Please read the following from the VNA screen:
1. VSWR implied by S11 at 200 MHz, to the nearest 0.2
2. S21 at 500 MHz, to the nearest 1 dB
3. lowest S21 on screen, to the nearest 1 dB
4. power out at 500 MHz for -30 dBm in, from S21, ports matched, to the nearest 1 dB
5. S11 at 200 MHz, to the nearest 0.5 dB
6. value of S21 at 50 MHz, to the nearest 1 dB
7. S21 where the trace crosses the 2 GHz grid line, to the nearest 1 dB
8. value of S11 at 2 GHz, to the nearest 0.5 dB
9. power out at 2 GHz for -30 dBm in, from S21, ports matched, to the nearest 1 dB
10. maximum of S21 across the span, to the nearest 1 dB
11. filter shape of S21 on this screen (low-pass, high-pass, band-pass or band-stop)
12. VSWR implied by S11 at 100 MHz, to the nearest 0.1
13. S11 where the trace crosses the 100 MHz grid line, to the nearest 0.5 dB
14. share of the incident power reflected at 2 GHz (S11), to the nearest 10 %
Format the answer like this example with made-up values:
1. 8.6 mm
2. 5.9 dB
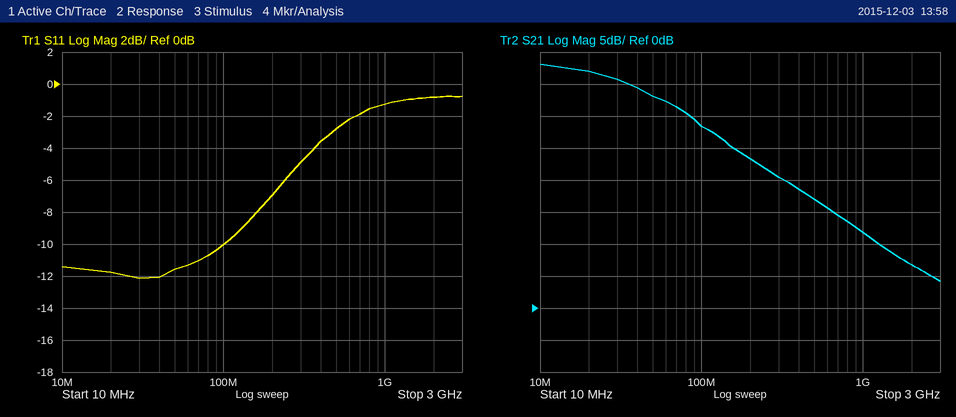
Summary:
1. 2.6
2. 17 dB
3. 4 dB
4. -13 dBm
5. -7.0 dB
6. 33 dB
7. 7 dB
8. -1.0 dB
9. -23 dBm
10. 38 dB
11. low-pass
12. 1.9
13. -10.0 dB
14. 80 %
